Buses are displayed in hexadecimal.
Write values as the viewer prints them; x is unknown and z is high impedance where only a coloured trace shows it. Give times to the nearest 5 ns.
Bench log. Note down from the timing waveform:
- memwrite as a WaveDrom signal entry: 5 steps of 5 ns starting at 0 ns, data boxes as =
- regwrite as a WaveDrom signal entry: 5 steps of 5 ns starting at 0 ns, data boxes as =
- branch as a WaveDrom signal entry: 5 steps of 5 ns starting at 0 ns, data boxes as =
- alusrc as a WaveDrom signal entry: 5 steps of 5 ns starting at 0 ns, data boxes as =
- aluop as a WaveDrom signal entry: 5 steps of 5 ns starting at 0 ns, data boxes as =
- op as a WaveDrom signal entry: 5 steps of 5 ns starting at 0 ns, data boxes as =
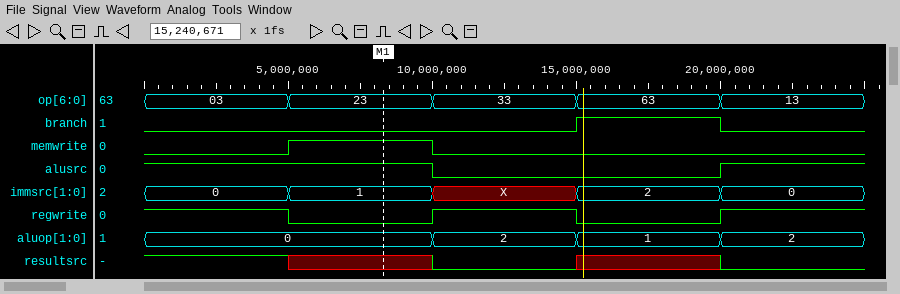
{name: 'memwrite', wave: '010..'}
{name: 'regwrite', wave: '10101'}
{name: 'branch', wave: '0..10'}
{name: 'alusrc', wave: '1.0.1'}
{name: 'aluop', wave: '=.===', data: '0 2 1 2'}
{name: 'op', wave: '=====', data: '03 23 33 63 13'}
